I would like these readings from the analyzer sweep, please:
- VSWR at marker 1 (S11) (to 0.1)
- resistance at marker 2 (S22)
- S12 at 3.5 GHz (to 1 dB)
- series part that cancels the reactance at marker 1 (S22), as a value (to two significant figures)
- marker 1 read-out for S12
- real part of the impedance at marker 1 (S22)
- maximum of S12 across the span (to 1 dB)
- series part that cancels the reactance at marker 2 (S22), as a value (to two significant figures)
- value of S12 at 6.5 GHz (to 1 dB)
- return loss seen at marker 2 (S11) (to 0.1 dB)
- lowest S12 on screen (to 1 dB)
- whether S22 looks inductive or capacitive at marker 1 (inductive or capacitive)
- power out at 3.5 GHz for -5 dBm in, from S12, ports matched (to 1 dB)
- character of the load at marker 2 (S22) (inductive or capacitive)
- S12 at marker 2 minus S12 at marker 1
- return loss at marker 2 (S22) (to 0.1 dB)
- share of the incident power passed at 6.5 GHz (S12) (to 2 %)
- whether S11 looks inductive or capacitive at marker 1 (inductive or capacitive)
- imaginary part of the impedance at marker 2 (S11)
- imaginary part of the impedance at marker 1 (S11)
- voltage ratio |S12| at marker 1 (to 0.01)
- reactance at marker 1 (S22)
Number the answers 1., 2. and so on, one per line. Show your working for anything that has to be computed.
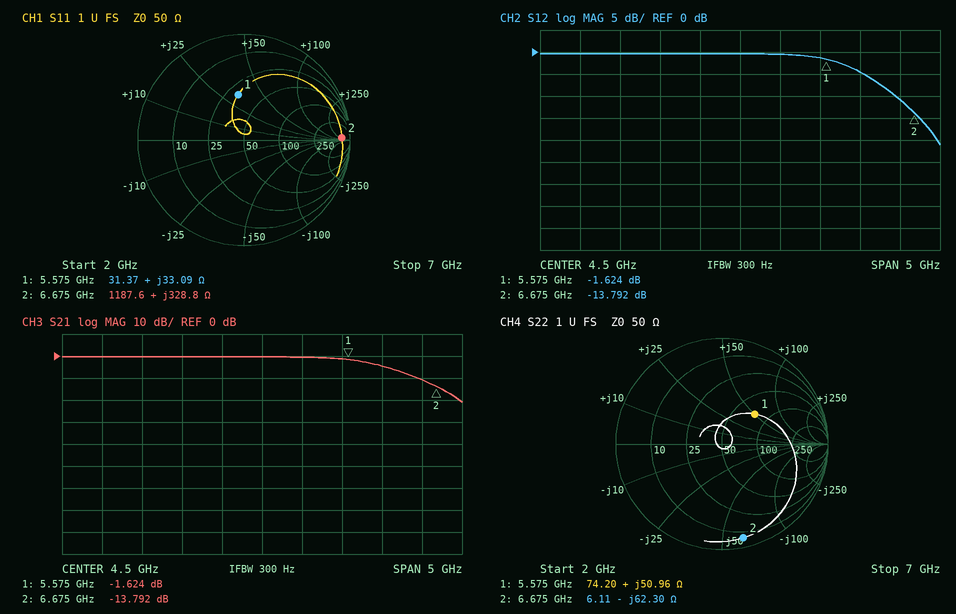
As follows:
1. 2.5
2. 6.11 Ω
3. 0 dB
4. C = 1/(2π × 5.575 GHz × 50.96 Ω) ≈ 560 fF
5. -1.624 dB
6. 74.20 Ω
7. 0 dB
8. L = 62.3 Ω/(2π × 6.675 GHz) ≈ 1.5 nH
9. -11 dB
10. 0.7 dB
11. -21 dB
12. inductive
13. -5 dBm + (0 dB) = -5 dBm
14. capacitive
15. -13.792 − (-1.624) = -12.168 dB
16. 0.8 dB
17. 10^(-11/10) ≈ 8 %
18. inductive
19. +328.8 Ω
20. +33.09 Ω
21. 10^(-1.624/20) ≈ 0.83
22. +50.96 Ω
